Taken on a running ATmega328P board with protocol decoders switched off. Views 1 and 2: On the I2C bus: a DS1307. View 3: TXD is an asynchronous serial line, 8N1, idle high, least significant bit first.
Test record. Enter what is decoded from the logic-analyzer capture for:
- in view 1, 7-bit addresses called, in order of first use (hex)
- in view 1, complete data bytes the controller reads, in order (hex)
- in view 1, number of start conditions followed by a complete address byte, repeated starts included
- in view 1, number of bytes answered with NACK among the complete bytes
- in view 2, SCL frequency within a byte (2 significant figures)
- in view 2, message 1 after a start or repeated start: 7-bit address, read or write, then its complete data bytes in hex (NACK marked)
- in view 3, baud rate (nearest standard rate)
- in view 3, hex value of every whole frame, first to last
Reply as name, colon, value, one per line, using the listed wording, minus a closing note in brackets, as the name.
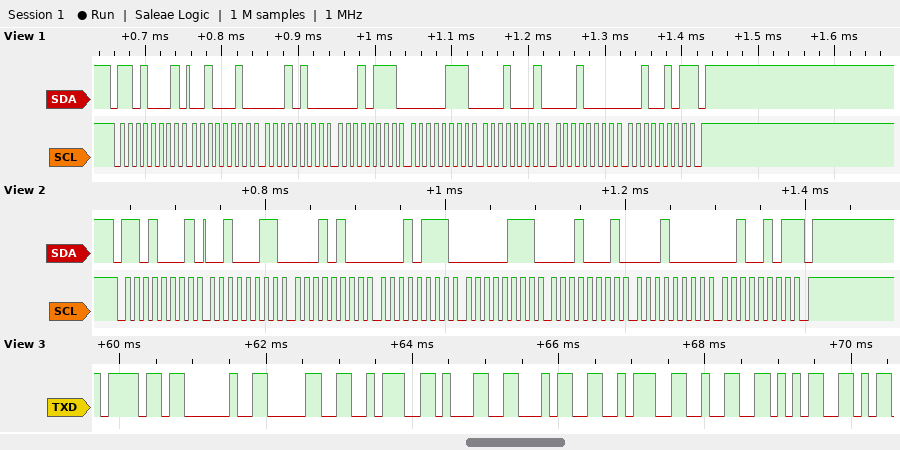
in view 1, 7-bit addresses called, in order of first use: 0x68
in view 1, complete data bytes the controller reads, in order: 22 14 17 07 11 10 25
in view 1, number of start conditions followed by a complete address byte, repeated starts included: 1
in view 1, number of bytes answered with NACK among the complete bytes: 1
in view 2, SCL frequency within a byte: 100 kHz
in view 2, message 1 after a start or repeated start: 7-bit address, read or write, then its complete data bytes in hex: 0x68 read: 23 14 17 07 11 10 25 NACK
in view 3, baud rate: 9600 baud
in view 3, hex value of every whole frame, first to last: 6F 20 30 3A 31 34 3A 32 35
